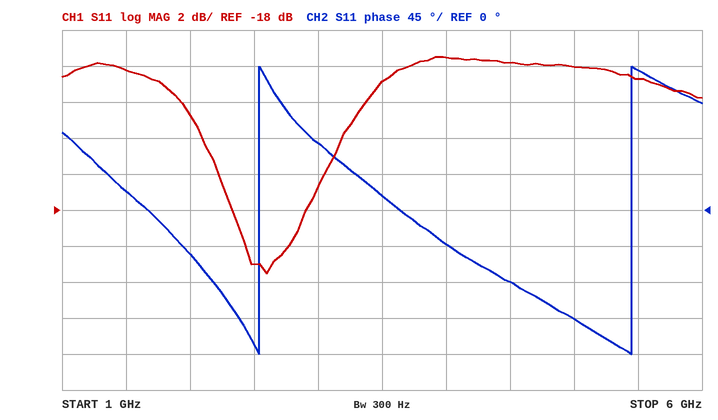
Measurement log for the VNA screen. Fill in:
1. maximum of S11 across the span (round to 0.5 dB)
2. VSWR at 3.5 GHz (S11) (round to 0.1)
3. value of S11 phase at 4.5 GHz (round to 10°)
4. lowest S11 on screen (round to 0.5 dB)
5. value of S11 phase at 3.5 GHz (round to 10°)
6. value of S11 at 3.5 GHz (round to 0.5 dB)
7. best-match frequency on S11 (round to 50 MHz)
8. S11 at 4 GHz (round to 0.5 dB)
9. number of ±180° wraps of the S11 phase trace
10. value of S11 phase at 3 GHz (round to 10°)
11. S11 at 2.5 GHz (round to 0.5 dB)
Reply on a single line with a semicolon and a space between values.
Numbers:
-9.5 dB; 1.8; -90°; -21.5 dB; 20°; -11.0 dB; 2.60 GHz; -9.5 dB; 2; 80°; -21.0 dB
